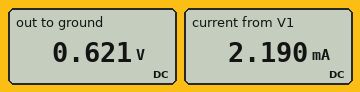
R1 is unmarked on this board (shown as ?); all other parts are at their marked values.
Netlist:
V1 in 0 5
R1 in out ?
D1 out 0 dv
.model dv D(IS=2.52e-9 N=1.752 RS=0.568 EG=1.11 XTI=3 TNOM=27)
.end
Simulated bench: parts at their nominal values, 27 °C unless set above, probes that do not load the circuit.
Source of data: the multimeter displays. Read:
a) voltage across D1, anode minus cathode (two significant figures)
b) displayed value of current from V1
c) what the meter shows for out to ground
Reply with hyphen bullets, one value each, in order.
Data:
- 620 mV
- 2.190 mA
- 0.621 V
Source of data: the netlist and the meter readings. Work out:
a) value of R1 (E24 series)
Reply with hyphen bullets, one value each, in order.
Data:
- 2 kΩ
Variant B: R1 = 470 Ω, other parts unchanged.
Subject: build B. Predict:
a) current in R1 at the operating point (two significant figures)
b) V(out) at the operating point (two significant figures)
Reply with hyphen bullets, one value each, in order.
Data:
- 9.2 mA
- 690 mV
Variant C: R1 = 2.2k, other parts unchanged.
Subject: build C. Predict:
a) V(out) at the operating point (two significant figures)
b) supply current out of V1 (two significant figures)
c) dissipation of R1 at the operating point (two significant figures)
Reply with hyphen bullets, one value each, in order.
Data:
- 620 mV
- 2.0 mA
- 8.7 mW
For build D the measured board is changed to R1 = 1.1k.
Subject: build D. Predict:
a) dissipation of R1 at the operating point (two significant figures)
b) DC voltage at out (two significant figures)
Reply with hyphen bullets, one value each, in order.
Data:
- 17 mW
- 650 mV
